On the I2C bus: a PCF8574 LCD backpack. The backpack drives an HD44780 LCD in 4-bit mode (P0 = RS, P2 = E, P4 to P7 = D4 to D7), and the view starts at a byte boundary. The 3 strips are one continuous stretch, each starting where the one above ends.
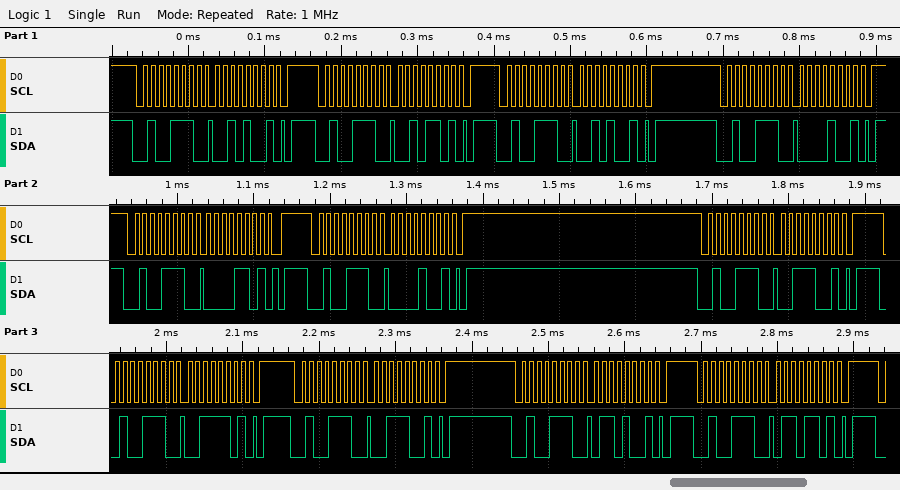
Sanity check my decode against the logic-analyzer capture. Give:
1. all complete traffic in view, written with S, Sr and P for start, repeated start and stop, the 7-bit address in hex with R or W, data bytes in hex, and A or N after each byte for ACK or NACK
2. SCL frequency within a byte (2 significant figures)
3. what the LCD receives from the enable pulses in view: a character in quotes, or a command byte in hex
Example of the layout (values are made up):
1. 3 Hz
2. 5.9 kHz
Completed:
1. S 27W A 29 A P S 27W A 2D A P S 27W A 29 A P S 27W A 09 A P S 27W A 0D A P S 27W A 09 A P S 27W A 39 A P S 27W A 3D A P S 27W A 39 A P S 27W A 69 A P S 27W A 6D A P
2. 100 kHz
3. ' '
